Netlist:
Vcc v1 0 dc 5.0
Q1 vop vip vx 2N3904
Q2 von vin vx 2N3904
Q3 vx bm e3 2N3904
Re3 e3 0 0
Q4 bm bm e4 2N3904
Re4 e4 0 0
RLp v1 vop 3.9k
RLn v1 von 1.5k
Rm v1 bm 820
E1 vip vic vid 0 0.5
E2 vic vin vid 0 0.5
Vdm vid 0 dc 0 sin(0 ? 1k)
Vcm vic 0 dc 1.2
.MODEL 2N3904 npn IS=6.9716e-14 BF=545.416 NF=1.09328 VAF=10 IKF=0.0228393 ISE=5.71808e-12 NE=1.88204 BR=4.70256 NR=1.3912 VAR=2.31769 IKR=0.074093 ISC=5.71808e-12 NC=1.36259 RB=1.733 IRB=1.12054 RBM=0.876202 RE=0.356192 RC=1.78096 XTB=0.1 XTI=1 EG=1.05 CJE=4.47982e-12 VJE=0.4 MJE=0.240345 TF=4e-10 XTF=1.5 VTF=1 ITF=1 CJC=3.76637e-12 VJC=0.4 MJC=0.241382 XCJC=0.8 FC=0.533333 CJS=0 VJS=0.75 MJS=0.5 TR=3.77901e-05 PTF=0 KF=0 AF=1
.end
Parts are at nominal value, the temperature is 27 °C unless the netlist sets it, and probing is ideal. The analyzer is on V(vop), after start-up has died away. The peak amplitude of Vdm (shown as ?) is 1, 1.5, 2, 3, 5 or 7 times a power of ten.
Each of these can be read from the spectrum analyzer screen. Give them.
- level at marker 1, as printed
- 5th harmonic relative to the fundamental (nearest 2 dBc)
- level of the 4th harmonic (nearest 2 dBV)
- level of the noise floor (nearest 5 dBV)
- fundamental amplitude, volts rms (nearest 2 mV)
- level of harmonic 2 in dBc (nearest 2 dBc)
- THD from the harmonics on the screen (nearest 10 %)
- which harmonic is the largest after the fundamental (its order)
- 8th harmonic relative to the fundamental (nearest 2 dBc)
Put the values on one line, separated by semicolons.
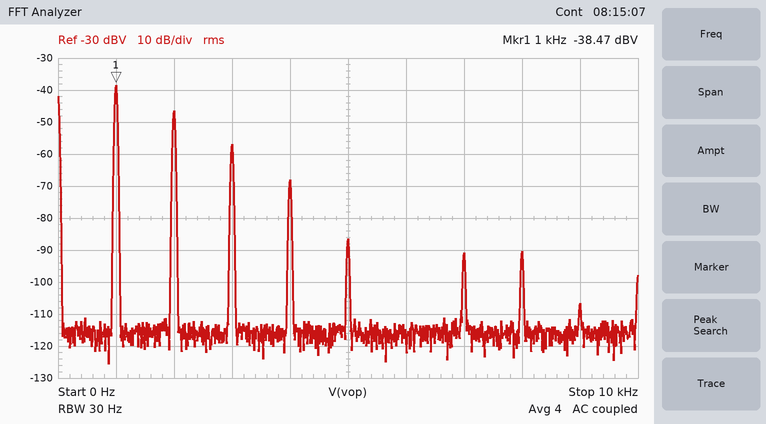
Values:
-38.47 dBV; -48 dBc; -68 dBV; -115 dBV; 12 mV; -8 dBc; 40 %; 2; -52 dBc
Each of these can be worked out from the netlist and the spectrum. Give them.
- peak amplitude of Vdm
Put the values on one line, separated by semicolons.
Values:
30 mV
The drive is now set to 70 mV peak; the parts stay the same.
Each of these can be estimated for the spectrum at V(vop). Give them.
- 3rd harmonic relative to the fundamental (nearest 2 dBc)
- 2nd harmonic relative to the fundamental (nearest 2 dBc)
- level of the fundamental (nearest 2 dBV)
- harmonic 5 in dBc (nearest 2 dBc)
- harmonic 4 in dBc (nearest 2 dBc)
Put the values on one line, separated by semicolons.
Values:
-8 dBc; -2 dBc; -6 dBV; -34 dBc; -16 dBc
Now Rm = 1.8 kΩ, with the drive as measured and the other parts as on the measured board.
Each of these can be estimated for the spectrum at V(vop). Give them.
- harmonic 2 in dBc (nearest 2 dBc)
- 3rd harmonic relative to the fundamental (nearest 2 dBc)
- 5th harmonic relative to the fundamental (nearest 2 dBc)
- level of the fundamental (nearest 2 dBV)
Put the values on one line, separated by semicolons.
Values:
-12 dBc; -22 dBc; -30 dBc; -2 dBV
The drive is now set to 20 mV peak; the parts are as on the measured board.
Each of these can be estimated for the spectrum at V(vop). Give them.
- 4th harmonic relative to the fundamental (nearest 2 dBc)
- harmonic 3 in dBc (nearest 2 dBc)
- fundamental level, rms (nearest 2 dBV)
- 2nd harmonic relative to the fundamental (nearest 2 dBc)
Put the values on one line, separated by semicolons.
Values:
-36 dBc; -24 dBc; -44 dBV; -12 dBc
